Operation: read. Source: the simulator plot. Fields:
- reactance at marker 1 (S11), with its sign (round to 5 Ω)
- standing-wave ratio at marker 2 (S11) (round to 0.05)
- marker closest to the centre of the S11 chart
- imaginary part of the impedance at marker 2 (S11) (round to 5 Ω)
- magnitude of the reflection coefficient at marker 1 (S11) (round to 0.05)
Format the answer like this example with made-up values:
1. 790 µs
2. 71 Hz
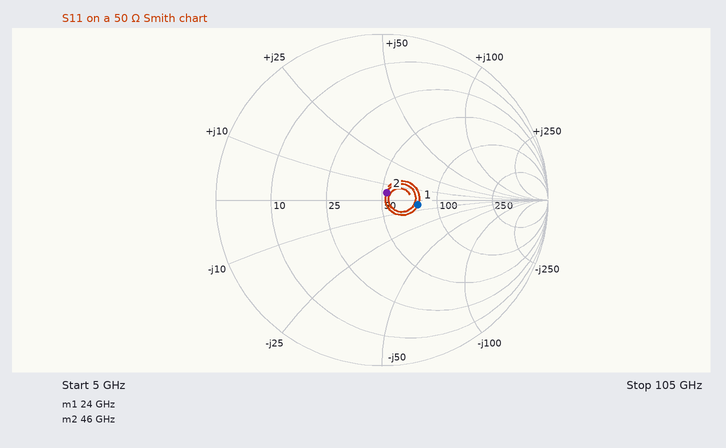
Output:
1. -5 Ω
2. 1.10
3. marker 2
4. +5 Ω
5. 0.20
